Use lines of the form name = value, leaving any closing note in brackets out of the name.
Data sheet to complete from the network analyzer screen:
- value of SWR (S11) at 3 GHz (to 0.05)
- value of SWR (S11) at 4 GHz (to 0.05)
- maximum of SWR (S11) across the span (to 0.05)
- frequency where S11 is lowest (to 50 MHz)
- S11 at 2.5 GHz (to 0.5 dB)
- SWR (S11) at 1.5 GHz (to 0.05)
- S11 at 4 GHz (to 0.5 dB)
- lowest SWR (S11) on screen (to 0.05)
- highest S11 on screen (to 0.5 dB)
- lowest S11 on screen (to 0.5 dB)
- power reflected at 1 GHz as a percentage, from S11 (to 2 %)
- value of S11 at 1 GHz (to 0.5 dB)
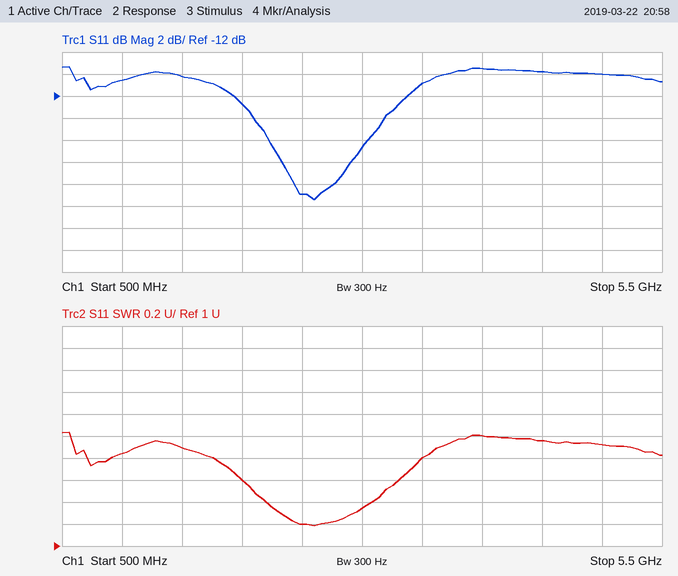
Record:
value of SWR (S11) at 3 GHz = 1.35
value of SWR (S11) at 4 GHz = 2.00
maximum of SWR (S11) across the span = 2.05
frequency where S11 is lowest = 2.60 GHz
S11 at 2.5 GHz = -21.0 dB
SWR (S11) at 1.5 GHz = 1.90
S11 at 4 GHz = -9.5 dB
lowest SWR (S11) on screen = 1.20
highest S11 on screen = -9.5 dB
lowest S11 on screen = -21.5 dB
power reflected at 1 GHz as a percentage, from S11 = 8 %
value of S11 at 1 GHz = -10.5 dB
